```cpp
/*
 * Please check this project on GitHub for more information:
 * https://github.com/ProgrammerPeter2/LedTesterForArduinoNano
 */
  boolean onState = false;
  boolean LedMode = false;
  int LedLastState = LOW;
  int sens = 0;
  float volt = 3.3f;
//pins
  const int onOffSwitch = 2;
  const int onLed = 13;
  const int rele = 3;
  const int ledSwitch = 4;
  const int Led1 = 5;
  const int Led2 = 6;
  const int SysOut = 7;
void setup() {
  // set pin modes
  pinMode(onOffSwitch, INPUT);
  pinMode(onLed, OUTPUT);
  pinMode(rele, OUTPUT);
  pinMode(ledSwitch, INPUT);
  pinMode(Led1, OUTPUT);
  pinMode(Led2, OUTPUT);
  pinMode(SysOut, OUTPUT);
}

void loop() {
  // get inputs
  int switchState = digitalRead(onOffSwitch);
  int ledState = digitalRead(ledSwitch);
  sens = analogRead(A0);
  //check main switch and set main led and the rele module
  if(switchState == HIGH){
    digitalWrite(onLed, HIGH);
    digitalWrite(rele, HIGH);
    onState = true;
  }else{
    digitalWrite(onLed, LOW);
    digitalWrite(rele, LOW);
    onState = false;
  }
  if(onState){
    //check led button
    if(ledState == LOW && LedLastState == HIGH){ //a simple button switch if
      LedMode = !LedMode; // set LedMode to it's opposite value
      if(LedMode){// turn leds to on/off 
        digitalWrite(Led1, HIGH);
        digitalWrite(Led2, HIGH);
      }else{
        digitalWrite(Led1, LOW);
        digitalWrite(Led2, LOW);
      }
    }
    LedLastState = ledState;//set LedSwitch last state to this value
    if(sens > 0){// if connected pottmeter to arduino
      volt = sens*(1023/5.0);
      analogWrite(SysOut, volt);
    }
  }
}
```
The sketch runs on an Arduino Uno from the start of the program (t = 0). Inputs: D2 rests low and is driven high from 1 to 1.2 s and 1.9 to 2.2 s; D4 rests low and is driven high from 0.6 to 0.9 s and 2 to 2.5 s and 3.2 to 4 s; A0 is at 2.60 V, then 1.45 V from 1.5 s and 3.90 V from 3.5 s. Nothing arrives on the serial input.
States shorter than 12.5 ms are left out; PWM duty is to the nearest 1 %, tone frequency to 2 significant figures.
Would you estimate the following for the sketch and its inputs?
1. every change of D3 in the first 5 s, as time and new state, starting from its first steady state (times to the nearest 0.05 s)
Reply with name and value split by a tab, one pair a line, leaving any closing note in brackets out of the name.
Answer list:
every change of D3 in the first 5 s, as time and new state, starting from its first steady state	0 s low; 1 s high; 1.2 s low; 1.9 s high; 2.2 s low
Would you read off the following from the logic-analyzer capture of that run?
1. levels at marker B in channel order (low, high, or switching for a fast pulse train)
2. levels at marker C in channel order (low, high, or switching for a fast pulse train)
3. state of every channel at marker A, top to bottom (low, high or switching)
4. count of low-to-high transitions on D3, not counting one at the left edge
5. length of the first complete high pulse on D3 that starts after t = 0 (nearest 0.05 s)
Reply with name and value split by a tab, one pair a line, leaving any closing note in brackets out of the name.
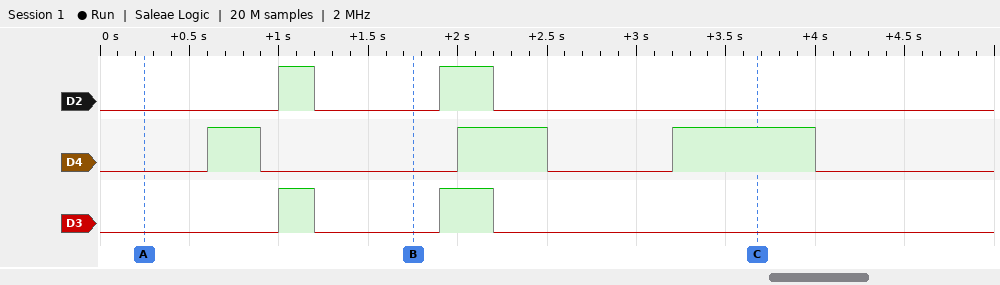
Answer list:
levels at marker B in channel order	D2 low, D4 low, D3 low
levels at marker C in channel order	D2 low, D4 high, D3 low
state of every channel at marker A, top to bottom	D2 low, D4 low, D3 low
count of low-to-high transitions on D3, not counting one at the left edge	2
length of the first complete high pulse on D3 that starts after t = 0	0.20 s
